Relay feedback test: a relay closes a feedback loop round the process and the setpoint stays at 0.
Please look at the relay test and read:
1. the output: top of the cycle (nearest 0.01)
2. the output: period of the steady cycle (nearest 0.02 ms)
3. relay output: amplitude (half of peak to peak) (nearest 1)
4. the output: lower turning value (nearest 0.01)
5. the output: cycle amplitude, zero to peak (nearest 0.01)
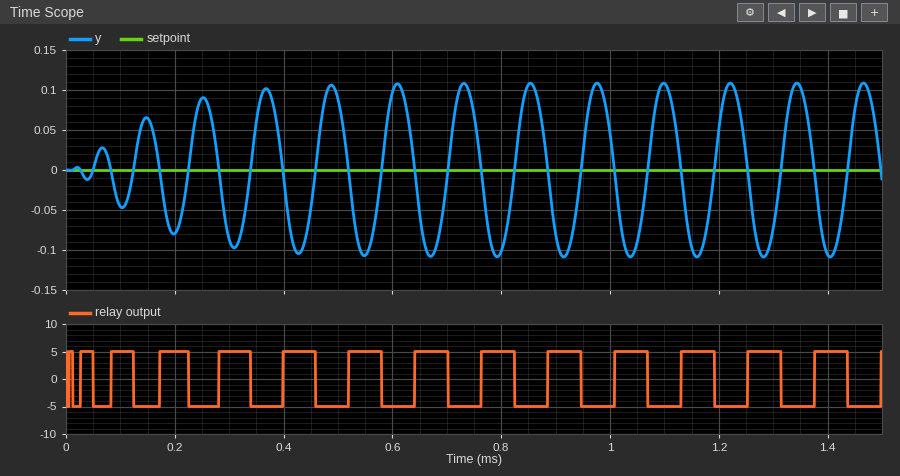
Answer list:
0.11
0.12 ms
5
-0.11
0.11
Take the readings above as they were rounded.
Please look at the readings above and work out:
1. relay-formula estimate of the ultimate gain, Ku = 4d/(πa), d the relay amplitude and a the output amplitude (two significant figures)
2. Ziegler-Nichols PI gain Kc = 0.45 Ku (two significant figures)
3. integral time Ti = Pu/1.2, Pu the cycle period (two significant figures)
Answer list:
58
26
0.10 ms
